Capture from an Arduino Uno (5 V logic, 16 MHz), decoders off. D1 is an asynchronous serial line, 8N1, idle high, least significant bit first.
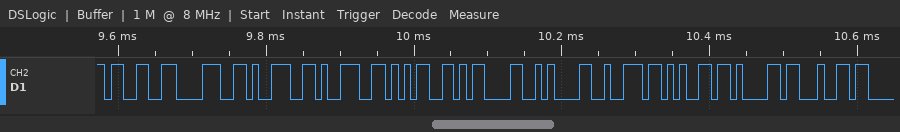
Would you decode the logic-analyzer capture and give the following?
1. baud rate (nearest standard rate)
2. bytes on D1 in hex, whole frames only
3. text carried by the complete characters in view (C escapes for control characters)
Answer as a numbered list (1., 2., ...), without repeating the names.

1. 115200 baud
2. 33 38 39 39 35 0D 0A 72 65 61 64
3. "38995\r\nread"
